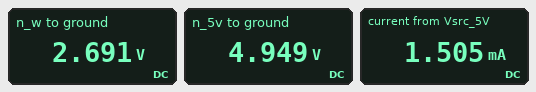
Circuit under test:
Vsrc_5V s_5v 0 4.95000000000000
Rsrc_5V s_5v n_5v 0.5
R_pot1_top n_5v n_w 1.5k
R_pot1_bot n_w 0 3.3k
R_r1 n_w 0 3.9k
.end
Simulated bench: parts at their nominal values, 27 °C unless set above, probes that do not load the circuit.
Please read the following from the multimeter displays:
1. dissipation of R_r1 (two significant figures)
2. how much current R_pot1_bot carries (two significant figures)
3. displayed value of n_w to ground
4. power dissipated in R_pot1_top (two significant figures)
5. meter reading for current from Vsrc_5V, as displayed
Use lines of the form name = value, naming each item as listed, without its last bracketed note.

dissipation of R_r1 = 1.9 mW
how much current R_pot1_bot carries = 820 µA
displayed value of n_w to ground = 2.691 V
power dissipated in R_pot1_top = 3.4 mW
meter reading for current from Vsrc_5V, as displayed = 1.505 mA
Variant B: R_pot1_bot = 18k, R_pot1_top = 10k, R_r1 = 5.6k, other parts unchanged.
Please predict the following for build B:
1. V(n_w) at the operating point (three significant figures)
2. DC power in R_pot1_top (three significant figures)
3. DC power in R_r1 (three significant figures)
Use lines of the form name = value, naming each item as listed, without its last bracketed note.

V(n_w) at the operating point = 1.48 V
DC power in R_pot1_top = 1.20 mW
DC power in R_r1 = 392 µW
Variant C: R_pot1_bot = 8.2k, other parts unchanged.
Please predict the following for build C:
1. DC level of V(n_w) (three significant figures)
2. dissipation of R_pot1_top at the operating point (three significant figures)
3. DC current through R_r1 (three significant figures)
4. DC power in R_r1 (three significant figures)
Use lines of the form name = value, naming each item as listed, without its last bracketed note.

DC level of V(n_w) = 3.16 V
dissipation of R_pot1_top at the operating point = 2.14 mW
DC current through R_r1 = 810 µA
DC power in R_r1 = 2.56 mW
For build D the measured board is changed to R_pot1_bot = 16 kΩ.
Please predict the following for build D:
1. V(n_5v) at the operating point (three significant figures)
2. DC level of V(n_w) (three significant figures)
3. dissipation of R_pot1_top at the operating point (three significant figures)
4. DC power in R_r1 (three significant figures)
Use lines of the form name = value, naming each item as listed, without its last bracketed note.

V(n_5v) at the operating point = 4.95 V
DC level of V(n_w) = 3.35 V
dissipation of R_pot1_top at the operating point = 1.71 mW
DC power in R_r1 = 2.87 mW
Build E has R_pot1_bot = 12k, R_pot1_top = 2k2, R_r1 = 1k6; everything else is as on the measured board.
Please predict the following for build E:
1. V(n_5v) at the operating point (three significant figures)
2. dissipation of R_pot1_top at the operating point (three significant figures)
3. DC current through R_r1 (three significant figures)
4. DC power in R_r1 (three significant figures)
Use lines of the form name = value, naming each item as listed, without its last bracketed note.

V(n_5v) at the operating point = 4.95 V
dissipation of R_pot1_top at the operating point = 4.13 mW
DC current through R_r1 = 1.21 mA
DC power in R_r1 = 2.34 mW
